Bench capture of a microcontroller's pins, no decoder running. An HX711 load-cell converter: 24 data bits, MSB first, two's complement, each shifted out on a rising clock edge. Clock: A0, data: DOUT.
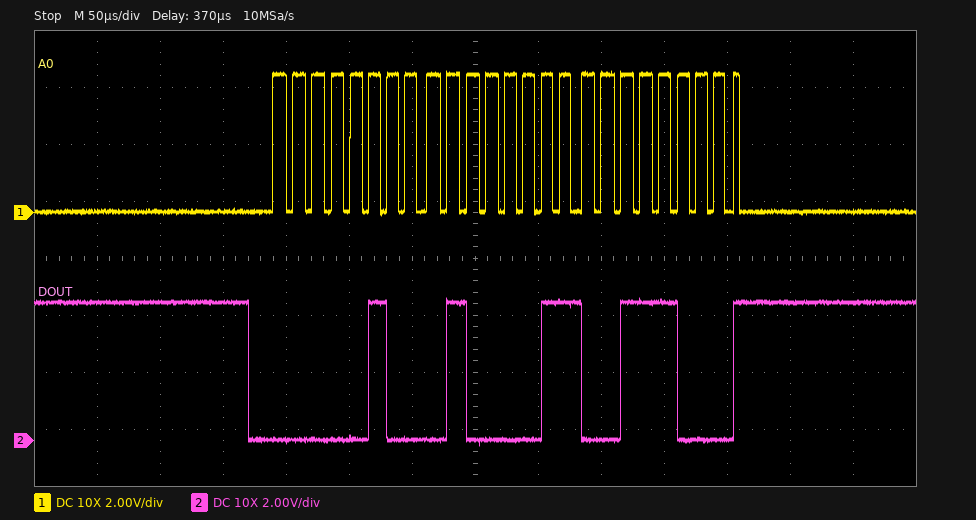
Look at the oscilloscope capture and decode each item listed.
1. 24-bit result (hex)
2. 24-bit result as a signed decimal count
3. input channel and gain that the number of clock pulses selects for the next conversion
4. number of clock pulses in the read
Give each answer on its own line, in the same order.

0x044338
279352
channel A, gain 128
25
